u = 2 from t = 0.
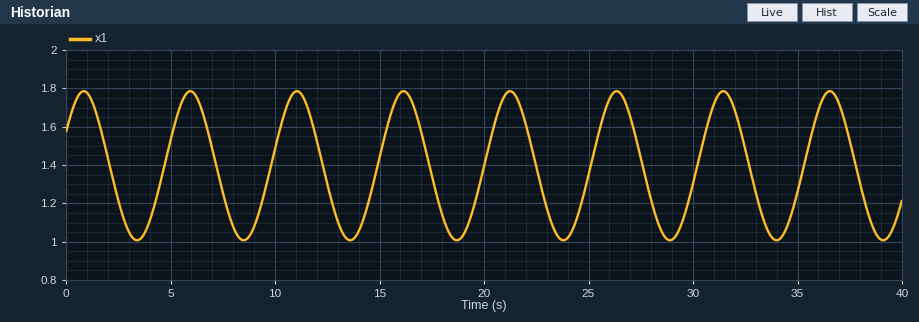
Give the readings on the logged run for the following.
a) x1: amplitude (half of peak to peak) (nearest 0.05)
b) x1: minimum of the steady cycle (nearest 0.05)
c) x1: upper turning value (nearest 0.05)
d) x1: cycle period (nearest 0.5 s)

0.40
1.00
1.80
5.0 s
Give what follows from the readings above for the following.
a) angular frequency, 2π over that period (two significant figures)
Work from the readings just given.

1.3 rad/s
